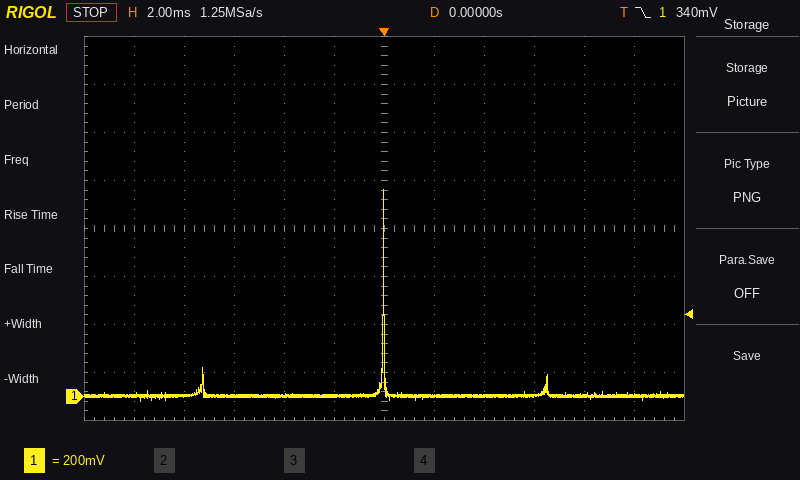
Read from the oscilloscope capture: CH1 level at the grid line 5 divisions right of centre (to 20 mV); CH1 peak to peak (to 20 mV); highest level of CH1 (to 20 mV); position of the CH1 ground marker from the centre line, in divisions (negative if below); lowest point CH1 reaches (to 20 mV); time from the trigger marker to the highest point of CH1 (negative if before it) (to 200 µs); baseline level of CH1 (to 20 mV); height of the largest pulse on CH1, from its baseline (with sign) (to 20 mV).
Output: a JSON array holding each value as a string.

["0 mV", "880 mV", "860 mV", "-3.5 div", "-20 mV", "0.0 ms", "0 mV", "+860 mV"]
